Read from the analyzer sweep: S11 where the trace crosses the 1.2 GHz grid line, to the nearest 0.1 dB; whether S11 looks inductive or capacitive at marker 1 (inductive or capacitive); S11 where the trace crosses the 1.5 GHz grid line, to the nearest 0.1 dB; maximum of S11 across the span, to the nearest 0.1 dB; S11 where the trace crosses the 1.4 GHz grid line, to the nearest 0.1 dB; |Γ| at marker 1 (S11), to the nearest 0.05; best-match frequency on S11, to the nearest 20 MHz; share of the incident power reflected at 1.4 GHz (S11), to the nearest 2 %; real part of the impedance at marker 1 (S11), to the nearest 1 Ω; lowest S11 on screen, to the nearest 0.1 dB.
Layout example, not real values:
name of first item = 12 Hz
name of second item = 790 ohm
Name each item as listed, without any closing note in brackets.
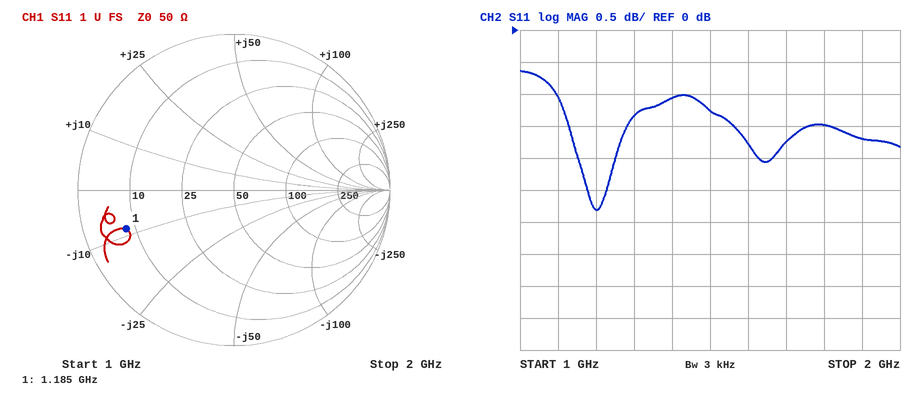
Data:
S11 where the trace crosses the 1.2 GHz grid line, to the nearest 0.1 dB = -2.8 dB
whether S11 looks inductive or capacitive at marker 1 = capacitive
S11 where the trace crosses the 1.5 GHz grid line, to the nearest 0.1 dB = -1.3 dB
maximum of S11 across the span, to the nearest 0.1 dB = -0.6 dB
S11 where the trace crosses the 1.4 GHz grid line, to the nearest 0.1 dB = -1.1 dB
|Γ| at marker 1 (S11), to the nearest 0.05 = 0.75
best-match frequency on S11, to the nearest 20 MHz = 1.20 GHz
share of the incident power reflected at 1.4 GHz (S11), to the nearest 2 % = 78 %
real part of the impedance at marker 1 (S11), to the nearest 1 Ω = 8 Ω
lowest S11 on screen, to the nearest 0.1 dB = -2.8 dB
